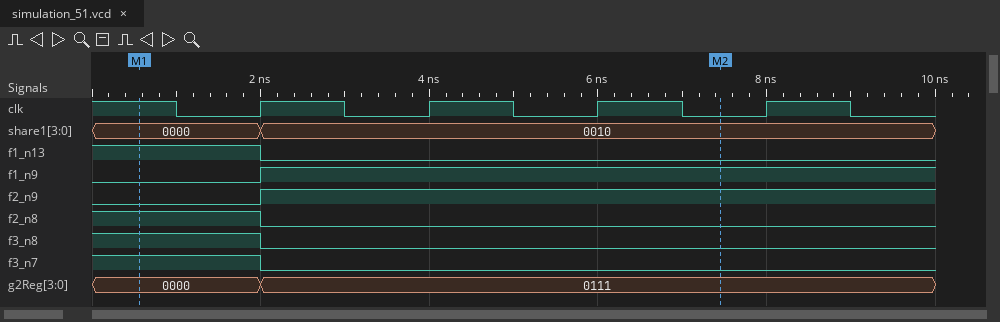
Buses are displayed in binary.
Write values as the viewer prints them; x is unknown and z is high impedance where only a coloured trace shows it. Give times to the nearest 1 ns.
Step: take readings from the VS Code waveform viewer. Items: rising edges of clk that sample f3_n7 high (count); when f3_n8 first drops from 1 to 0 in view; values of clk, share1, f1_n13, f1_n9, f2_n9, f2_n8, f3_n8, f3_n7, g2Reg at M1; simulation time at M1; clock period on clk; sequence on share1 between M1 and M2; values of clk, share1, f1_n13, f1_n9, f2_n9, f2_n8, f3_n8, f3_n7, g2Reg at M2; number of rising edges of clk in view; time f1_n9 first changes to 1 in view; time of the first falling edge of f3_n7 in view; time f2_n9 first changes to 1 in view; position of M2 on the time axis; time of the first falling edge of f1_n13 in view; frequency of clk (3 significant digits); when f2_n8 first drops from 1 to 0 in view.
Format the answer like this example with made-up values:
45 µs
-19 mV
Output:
1
2 ns
clk=1, share1=0000, f1_n13=1, f1_n9=0, f2_n9=0, f2_n8=1, f3_n8=1, f3_n7=1, g2Reg=0000
1 ns
2 ns
0000, 0010
clk=0, share1=0010, f1_n13=0, f1_n9=1, f2_n9=1, f2_n8=0, f3_n8=0, f3_n7=0, g2Reg=0111
4
2 ns
2 ns
2 ns
7 ns
2 ns
500 MHz
2 ns
